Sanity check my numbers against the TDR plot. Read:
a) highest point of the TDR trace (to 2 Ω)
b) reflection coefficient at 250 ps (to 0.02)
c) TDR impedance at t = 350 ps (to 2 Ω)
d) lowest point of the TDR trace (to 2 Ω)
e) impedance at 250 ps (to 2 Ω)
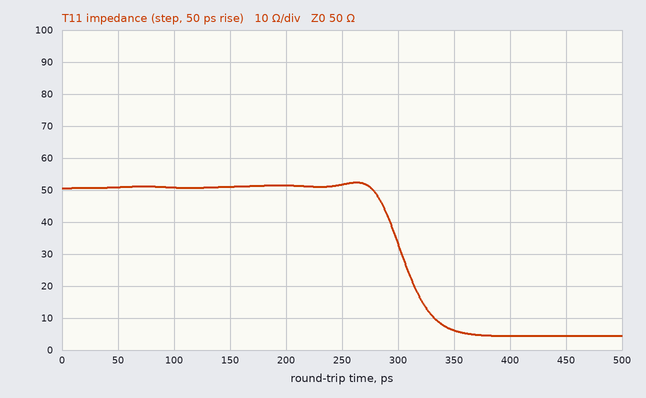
52 Ω
+0.02
6 Ω
4 Ω
52 Ω
